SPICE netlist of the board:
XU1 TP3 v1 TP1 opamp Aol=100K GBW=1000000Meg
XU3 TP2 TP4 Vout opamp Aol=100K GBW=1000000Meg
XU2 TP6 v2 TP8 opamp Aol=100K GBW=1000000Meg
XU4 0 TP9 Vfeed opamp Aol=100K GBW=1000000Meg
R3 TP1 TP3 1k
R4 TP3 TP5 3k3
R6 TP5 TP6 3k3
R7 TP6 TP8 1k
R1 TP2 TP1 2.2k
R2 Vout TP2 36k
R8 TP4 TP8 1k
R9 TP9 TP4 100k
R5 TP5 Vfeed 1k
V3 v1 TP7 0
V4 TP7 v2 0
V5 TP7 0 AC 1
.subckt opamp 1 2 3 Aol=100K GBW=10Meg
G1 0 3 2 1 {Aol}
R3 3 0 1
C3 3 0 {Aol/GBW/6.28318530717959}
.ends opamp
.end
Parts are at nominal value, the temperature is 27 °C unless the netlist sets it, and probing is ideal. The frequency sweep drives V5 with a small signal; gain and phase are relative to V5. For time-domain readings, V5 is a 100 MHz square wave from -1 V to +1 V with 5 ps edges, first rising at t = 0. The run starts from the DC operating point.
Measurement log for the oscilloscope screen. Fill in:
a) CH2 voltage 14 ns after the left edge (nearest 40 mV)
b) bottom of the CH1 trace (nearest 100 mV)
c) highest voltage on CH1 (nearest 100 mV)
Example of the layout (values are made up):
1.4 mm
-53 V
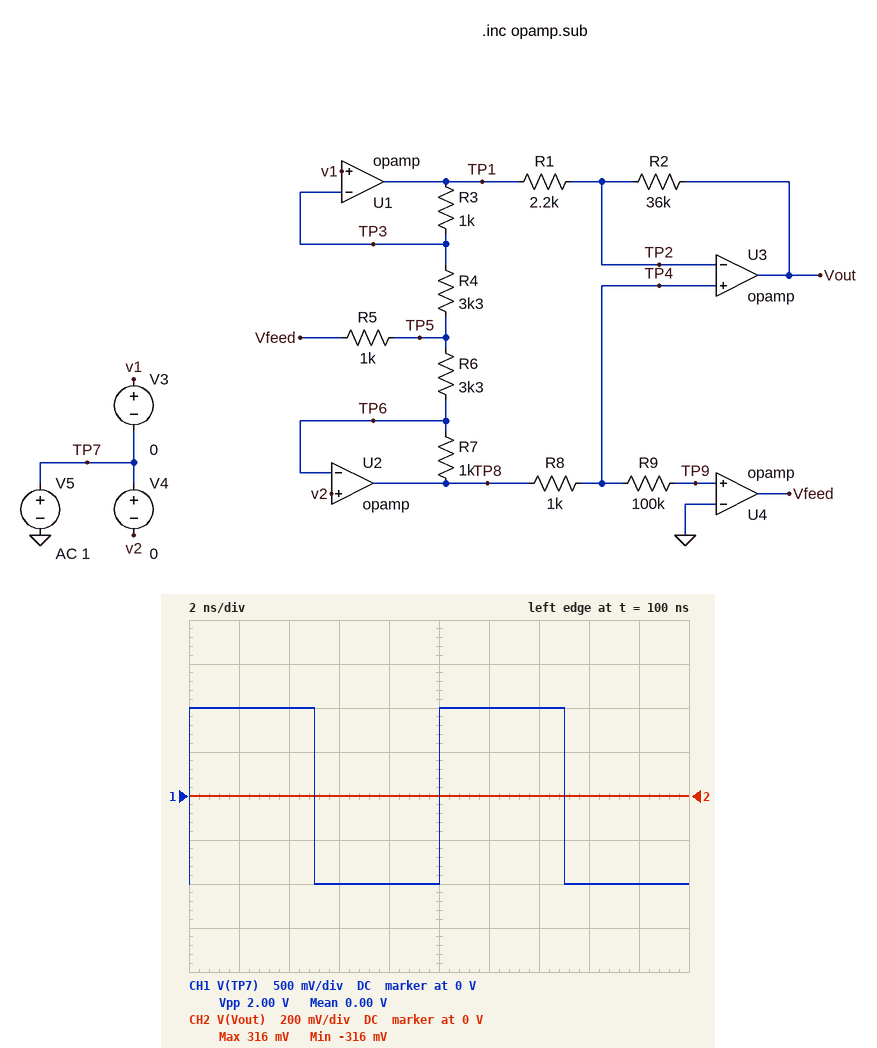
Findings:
0 V
-1.0 V
1.0 V
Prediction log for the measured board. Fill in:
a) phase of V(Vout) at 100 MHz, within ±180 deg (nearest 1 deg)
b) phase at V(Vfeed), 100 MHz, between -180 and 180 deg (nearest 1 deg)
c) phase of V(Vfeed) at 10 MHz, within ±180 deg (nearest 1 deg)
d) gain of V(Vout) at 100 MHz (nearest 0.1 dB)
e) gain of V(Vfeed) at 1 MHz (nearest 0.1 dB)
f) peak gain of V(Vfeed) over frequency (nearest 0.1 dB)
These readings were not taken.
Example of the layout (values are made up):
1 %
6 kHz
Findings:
84 deg
0 deg
0 deg
-64.0 dB
16.0 dB
16.0 dB
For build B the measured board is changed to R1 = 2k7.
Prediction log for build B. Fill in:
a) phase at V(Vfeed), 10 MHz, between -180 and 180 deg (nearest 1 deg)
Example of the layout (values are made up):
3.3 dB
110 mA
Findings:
0 deg
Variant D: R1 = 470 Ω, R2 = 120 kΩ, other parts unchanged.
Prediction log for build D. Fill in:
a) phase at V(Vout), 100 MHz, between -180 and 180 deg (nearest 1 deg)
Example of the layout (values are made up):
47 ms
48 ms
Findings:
83 deg
